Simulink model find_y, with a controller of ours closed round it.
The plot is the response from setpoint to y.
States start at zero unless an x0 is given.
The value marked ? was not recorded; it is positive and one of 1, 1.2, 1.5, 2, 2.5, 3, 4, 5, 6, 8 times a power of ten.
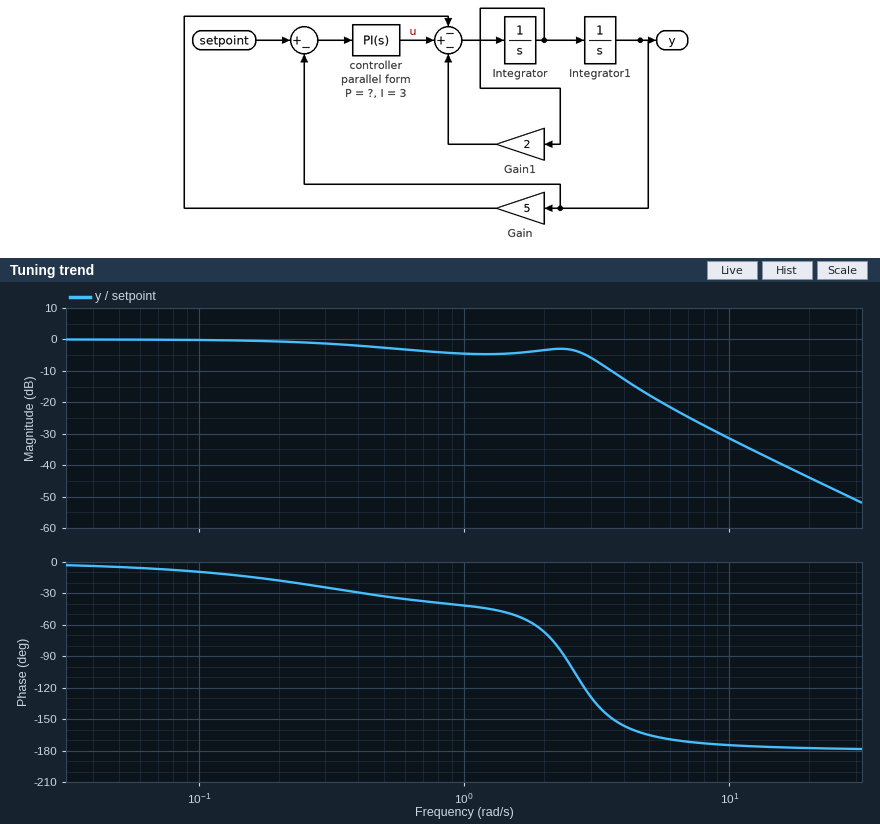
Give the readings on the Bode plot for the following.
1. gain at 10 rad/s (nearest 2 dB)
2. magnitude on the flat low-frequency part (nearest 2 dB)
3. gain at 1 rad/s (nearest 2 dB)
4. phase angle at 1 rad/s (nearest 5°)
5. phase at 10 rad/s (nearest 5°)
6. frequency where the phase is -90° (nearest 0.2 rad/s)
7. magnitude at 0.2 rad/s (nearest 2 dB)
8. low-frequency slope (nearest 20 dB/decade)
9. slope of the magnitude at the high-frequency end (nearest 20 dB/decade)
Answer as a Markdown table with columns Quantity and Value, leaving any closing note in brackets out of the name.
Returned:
| Quantity | Value |
|---|---|
| gain at 10 rad/s | -32 dB |
| magnitude on the flat low-frequency part | 0 dB |
| gain at 1 rad/s | -4 dB |
| phase angle at 1 rad/s | -40° |
| phase at 10 rad/s | -175° |
| frequency where the phase is -90° | 2.4 rad/s |
| magnitude at 0.2 rad/s | 0 dB |
| low-frequency slope | 0 dB/decade |
| slope of the magnitude at the high-frequency end | -40 dB/decade |
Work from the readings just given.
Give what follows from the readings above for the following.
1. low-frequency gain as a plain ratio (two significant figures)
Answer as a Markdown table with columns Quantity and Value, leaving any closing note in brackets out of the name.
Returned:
| Quantity | Value |
|---|---|
| low-frequency gain as a plain ratio | 1.0 |
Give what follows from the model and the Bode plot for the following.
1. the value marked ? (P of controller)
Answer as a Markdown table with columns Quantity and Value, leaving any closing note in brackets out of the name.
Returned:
| Quantity | Value |
|---|---|
| the value marked ? | 2.5 |
